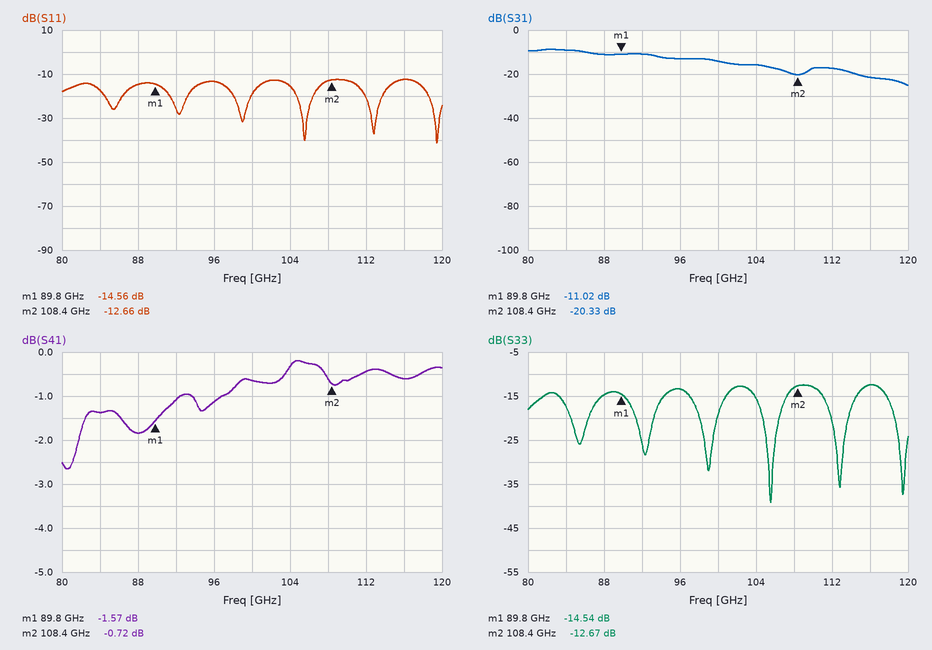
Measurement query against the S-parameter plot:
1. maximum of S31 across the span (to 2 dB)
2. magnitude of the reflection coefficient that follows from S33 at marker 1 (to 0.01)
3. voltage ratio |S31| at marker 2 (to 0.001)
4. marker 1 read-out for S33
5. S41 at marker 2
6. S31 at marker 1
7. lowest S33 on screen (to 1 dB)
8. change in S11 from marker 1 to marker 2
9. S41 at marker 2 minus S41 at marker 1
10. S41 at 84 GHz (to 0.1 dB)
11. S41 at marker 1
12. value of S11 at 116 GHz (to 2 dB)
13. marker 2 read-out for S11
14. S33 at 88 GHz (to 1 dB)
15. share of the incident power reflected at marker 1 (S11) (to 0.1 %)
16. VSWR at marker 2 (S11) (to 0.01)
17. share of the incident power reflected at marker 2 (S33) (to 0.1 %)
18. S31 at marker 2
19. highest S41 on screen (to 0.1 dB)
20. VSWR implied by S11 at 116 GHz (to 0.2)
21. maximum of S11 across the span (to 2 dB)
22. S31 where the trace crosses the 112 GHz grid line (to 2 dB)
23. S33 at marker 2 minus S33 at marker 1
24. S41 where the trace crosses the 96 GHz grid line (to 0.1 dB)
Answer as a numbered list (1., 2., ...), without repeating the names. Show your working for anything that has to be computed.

1. -8 dB
2. 10^(-14.54/20) ≈ 0.19
3. 10^(-20.33/20) ≈ 0.096
4. -14.54 dB
5. -0.72 dB
6. -11.02 dB
7. -39 dB
8. -12.66 − (-14.56) = 1.90 dB
9. -0.72 − (-1.57) = 0.85 dB
10. -1.4 dB
11. -1.57 dB
12. -12 dB
13. -12.66 dB
14. -15 dB
15. 10^(-14.56/10) ≈ 3.5 %
16. (1 + 0.2328)/(1 − 0.2328) ≈ 1.61
17. 10^(-12.67/10) ≈ 5.4 %
18. -20.33 dB
19. -0.2 dB
20. |Γ| = 10^(-12/20) = 0.2512; VSWR = (1 + 0.2512)/(1 − 0.2512) ≈ 1.67, so 1.6 to the nearest 0.2
21. -12 dB
22. -18 dB
23. -12.67 − (-14.54) = 1.87 dB
24. -1.1 dB
